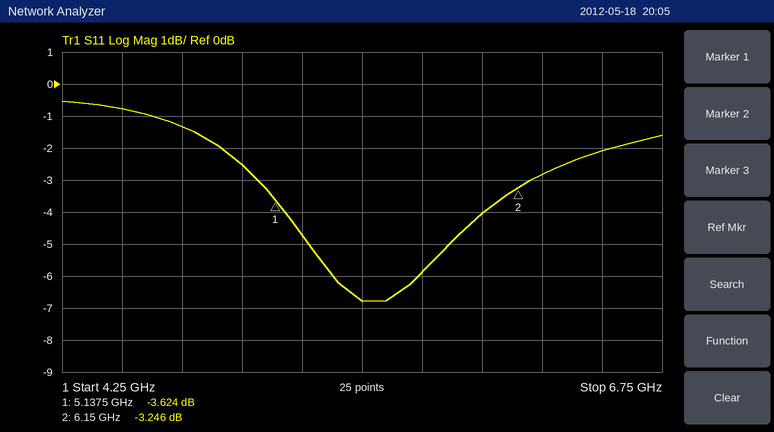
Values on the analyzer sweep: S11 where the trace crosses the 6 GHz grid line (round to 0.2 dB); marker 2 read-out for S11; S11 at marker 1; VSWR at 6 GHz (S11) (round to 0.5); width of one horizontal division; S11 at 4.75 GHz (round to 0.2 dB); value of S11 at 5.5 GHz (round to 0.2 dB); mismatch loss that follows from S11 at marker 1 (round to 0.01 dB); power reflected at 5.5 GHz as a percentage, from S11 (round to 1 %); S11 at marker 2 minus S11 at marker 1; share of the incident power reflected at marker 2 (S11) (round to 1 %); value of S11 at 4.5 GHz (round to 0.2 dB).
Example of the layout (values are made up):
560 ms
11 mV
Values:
-4.0 dB
-3.246 dB
-3.624 dB
4.5
250 MHz
-1.4 dB
-6.8 dB
2.47 dB
21 %
0.378 dB
47 %
-0.8 dB
